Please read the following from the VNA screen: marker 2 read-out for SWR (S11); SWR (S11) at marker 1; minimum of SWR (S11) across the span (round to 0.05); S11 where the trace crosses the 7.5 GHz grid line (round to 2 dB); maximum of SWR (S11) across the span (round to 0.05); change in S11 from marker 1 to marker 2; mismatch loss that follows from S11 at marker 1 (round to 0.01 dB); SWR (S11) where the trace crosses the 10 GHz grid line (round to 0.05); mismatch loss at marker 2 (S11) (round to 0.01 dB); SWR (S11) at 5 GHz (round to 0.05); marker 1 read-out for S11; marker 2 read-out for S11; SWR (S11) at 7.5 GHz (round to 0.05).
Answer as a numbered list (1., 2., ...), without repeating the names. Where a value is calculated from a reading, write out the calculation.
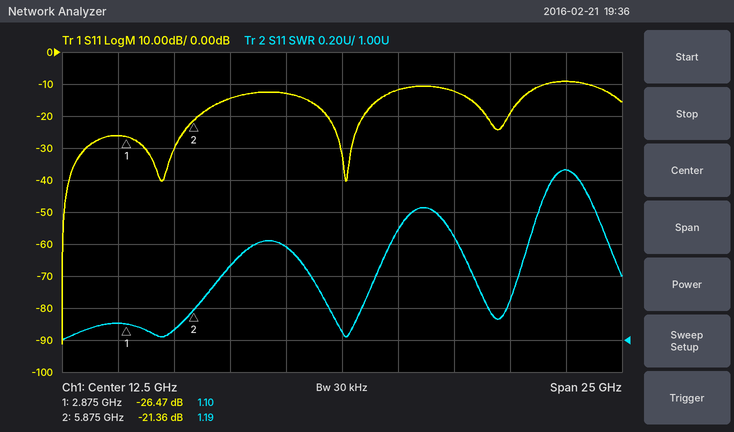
1. 1.19
2. 1.10
3. 1.00
4. -14 dB
5. 2.05
6. -21.36 − (-26.47) = 5.11 dB
7. −10 log10(1 − 10^(-26.47/10)) ≈ 0.01 dB
8. 1.60
9. −10 log10(1 − 10^(-21.36/10)) ≈ 0.03 dB
10. 1.05
11. -26.47 dB
12. -21.36 dB
13. 1.45
